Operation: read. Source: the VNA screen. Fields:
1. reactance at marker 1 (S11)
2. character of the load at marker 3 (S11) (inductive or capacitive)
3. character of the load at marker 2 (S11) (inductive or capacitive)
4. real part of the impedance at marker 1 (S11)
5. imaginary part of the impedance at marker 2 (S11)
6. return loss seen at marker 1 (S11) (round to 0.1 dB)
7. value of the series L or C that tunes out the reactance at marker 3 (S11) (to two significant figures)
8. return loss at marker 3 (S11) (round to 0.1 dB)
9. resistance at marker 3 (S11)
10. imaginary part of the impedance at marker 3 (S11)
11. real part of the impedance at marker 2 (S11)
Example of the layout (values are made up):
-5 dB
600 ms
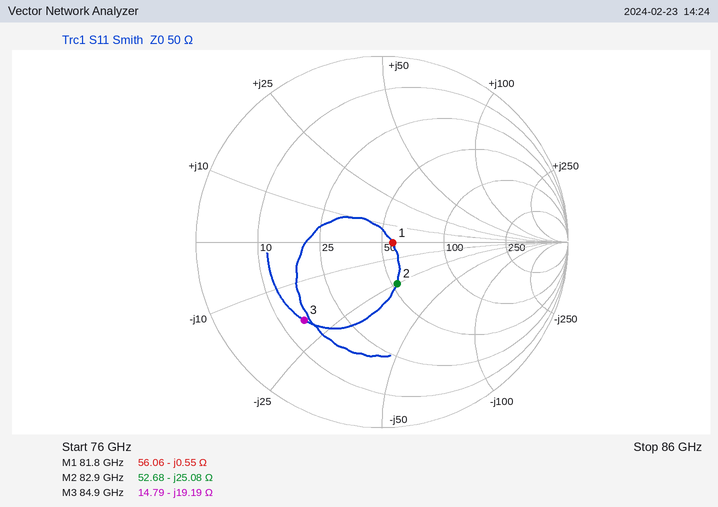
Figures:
-0.55 Ω
capacitive
capacitive
56.06 Ω
-25.08 Ω
24.8 dB
36 pH
4.5 dB
14.79 Ω
-19.19 Ω
52.68 Ω
